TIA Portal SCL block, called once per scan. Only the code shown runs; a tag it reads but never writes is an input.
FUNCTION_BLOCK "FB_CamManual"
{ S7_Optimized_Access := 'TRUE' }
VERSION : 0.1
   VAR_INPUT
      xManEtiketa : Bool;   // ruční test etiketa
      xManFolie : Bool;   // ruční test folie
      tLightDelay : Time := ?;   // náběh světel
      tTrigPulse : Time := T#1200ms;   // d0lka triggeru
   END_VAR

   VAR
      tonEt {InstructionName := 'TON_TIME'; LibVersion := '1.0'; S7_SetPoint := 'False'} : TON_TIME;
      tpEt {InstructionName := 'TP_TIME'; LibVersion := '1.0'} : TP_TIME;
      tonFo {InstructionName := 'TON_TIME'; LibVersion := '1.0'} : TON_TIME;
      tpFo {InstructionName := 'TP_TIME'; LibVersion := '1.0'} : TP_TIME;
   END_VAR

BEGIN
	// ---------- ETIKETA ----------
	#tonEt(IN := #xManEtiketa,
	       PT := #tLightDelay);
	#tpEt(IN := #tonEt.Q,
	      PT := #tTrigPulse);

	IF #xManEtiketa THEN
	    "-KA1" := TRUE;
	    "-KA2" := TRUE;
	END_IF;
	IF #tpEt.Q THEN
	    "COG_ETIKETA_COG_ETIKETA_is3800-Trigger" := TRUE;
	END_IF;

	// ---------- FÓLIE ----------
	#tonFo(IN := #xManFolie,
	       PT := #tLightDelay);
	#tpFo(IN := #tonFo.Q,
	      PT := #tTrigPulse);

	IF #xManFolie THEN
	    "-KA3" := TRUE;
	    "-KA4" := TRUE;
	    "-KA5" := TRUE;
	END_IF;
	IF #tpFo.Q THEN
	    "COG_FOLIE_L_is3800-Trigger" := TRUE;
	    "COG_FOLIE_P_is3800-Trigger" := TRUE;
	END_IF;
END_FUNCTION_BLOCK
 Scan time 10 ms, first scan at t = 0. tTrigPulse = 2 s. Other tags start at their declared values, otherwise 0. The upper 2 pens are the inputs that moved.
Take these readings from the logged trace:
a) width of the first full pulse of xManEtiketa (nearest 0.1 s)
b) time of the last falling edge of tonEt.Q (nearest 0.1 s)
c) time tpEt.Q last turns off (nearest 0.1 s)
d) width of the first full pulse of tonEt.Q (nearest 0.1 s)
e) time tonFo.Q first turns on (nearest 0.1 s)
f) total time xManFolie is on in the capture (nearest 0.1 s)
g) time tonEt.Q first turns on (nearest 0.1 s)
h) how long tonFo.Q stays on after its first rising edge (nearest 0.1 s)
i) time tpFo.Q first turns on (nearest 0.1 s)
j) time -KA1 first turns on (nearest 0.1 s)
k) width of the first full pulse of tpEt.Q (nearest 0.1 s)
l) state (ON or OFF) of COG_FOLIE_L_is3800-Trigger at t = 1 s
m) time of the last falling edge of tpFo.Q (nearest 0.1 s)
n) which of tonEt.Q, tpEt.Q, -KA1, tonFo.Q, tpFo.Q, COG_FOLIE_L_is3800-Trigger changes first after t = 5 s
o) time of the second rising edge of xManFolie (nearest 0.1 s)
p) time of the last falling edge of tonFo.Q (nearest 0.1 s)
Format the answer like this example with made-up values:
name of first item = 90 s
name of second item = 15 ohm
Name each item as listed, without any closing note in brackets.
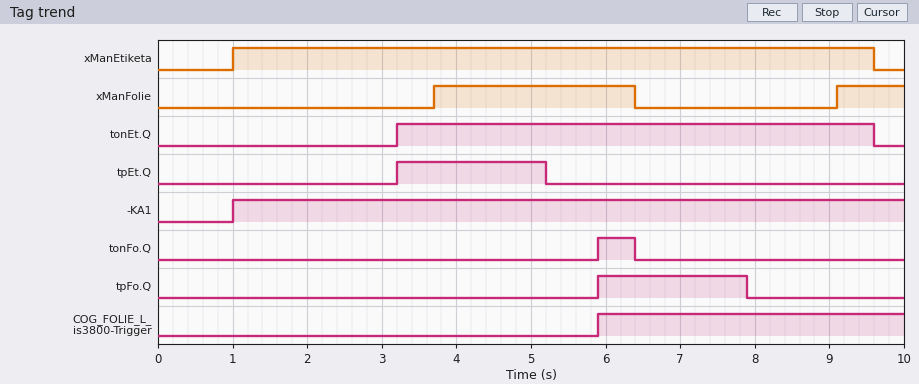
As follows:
width of the first full pulse of xManEtiketa = 8.6 s
time of the last falling edge of tonEt.Q = 9.6 s
time tpEt.Q last turns off = 5.2 s
width of the first full pulse of tonEt.Q = 6.4 s
time tonFo.Q first turns on = 5.9 s
total time xManFolie is on in the capture = 3.6 s
time tonEt.Q first turns on = 3.2 s
how long tonFo.Q stays on after its first rising edge = 0.5 s
time tpFo.Q first turns on = 5.9 s
time -KA1 first turns on = 1.0 s
width of the first full pulse of tpEt.Q = 2.0 s
state (ON or OFF) of COG_FOLIE_L_is3800-Trigger at t = 1 s = OFF
time of the last falling edge of tpFo.Q = 7.9 s
which of tonEt.Q, tpEt.Q, -KA1, tonFo.Q, tpFo.Q, COG_FOLIE_L_is3800-Trigger changes first after t = 5 s = tpEt.Q
time of the second rising edge of xManFolie = 9.1 s
time of the last falling edge of tonFo.Q = 6.4 s
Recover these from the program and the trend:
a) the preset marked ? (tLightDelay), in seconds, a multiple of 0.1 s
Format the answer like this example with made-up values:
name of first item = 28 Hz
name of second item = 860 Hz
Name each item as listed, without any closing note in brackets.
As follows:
the preset marked ? (tLightDelay), in seconds, a multiple of 0.1 s = 2.2 s
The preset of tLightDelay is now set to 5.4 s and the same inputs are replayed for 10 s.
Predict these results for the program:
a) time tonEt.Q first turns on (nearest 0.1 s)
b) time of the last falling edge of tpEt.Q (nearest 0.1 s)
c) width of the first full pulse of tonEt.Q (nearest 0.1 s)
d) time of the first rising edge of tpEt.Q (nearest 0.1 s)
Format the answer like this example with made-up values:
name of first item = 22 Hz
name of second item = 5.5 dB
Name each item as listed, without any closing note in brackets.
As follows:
time tonEt.Q first turns on = 6.4 s
time of the last falling edge of tpEt.Q = 8.4 s
width of the first full pulse of tonEt.Q = 3.2 s
time of the first rising edge of tpEt.Q = 6.4 s
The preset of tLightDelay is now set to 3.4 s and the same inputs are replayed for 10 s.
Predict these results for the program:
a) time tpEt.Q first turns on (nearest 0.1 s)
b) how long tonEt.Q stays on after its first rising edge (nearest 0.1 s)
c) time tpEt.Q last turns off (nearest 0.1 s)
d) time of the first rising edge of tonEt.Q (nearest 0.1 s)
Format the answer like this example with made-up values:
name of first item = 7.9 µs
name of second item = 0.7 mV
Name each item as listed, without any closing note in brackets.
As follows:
time tpEt.Q first turns on = 4.4 s
how long tonEt.Q stays on after its first rising edge = 5.2 s
time tpEt.Q last turns off = 6.4 s
time of the first rising edge of tonEt.Q = 4.4 s
